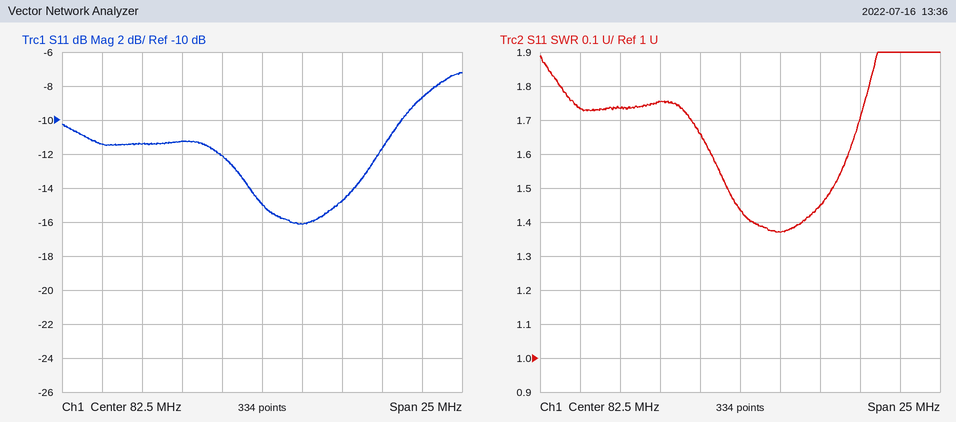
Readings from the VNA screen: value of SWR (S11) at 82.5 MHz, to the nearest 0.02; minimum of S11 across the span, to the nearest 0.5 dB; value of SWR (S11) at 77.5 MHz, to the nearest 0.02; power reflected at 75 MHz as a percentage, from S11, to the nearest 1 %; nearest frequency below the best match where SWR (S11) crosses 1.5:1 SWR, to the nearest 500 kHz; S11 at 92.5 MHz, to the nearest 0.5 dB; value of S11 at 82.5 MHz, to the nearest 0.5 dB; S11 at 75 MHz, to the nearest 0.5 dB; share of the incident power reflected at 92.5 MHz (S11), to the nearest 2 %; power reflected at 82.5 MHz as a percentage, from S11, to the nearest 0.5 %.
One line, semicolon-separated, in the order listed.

1.44; -16.0 dB; 1.76; 7 %; 81.5 MHz; -8.5 dB; -15.0 dB; -11.5 dB; 14 %; 3.0 %
